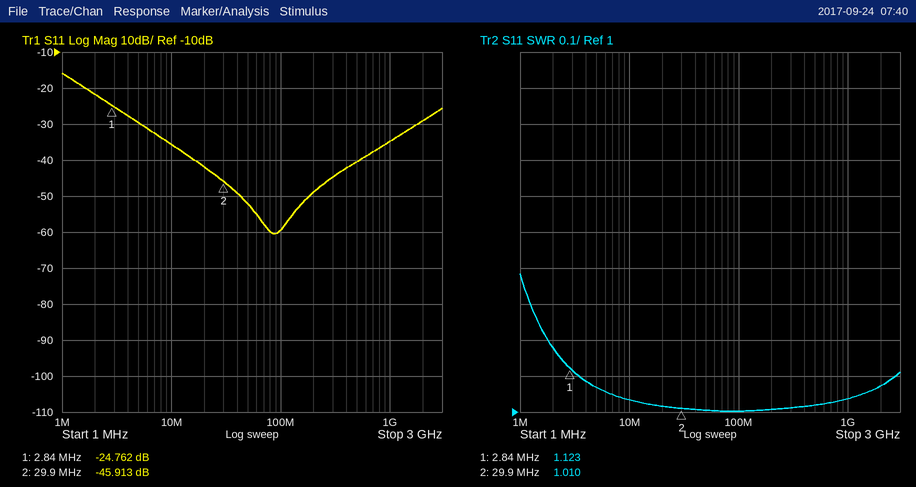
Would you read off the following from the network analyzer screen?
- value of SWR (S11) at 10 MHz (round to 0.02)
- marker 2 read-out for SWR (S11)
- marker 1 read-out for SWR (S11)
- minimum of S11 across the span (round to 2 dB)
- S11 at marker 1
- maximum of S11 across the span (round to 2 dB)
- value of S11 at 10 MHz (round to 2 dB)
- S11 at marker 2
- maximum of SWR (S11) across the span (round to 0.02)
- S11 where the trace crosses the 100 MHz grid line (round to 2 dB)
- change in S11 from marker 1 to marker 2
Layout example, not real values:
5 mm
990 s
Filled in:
1.04
1.010
1.123
-60 dB
-24.762 dB
-16 dB
-36 dB
-45.913 dB
1.38
-60 dB
-21.151 dB
